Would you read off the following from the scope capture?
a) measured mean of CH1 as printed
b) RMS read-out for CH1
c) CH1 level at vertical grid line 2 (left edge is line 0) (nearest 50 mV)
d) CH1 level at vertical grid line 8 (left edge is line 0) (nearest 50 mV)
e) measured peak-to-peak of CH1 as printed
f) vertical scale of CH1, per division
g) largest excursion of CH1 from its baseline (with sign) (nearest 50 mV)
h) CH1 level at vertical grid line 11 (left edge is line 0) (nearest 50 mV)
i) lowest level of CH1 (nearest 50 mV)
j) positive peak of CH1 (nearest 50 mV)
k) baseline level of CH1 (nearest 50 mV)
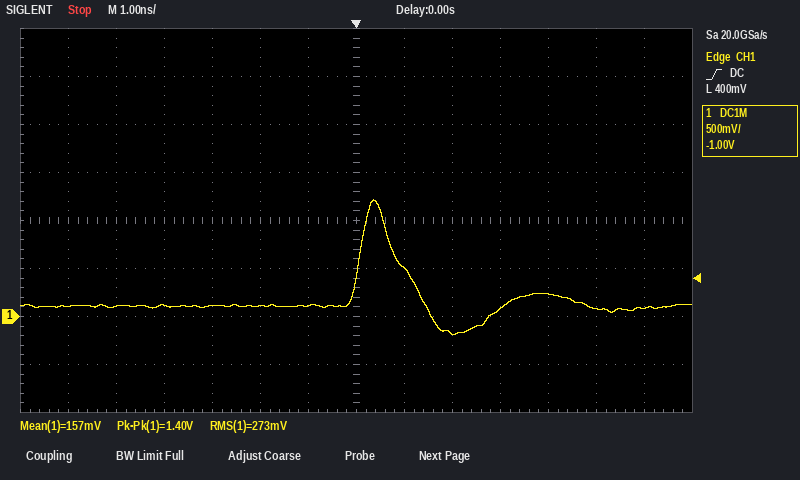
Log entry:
157 mV
273 mV
100 mV
500 mV
1.40 V
500 mV
+1.10 V
250 mV
-200 mV
1.20 V
100 mV
